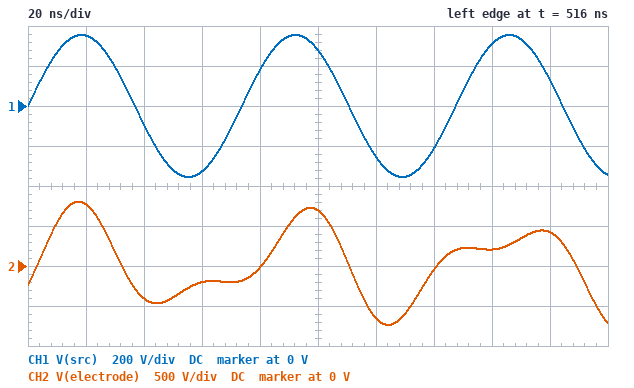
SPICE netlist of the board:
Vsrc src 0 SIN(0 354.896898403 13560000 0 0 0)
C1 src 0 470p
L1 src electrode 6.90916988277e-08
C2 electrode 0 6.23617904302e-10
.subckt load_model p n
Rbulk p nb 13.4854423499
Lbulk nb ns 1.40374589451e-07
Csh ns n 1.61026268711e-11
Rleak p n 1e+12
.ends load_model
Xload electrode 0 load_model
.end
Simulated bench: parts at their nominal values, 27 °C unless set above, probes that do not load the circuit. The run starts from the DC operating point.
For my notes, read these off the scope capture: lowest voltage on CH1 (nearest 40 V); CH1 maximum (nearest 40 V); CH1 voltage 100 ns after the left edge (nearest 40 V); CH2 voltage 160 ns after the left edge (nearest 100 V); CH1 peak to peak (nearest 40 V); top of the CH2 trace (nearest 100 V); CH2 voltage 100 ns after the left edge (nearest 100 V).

-360 V
360 V
280 V
200 V
720 V
800 V
700 V
